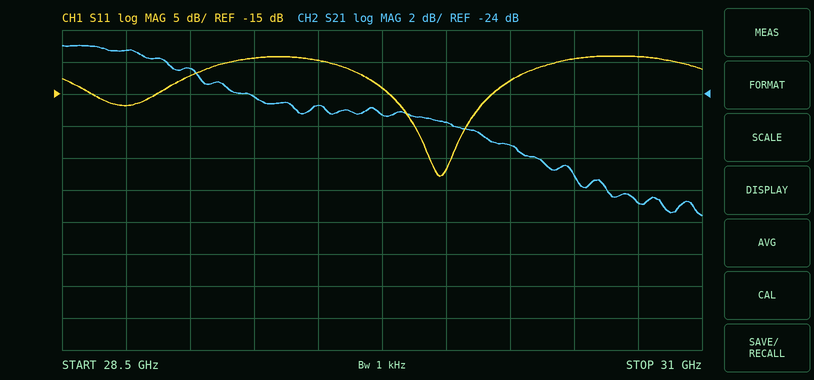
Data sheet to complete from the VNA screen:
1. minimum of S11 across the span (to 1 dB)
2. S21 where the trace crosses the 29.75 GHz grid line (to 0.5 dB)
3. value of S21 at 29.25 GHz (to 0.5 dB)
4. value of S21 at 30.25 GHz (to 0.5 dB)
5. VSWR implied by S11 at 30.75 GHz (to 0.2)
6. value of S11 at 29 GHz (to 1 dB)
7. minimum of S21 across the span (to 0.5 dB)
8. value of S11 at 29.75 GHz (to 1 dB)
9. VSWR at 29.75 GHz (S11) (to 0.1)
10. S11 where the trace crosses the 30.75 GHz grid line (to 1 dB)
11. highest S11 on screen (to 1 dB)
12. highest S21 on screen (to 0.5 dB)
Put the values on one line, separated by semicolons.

-28 dB; -25.5 dB; -24.0 dB; -27.0 dB; 2.0; -12 dB; -31.5 dB; -14 dB; 1.5; -9 dB; -9 dB; -21.0 dB
